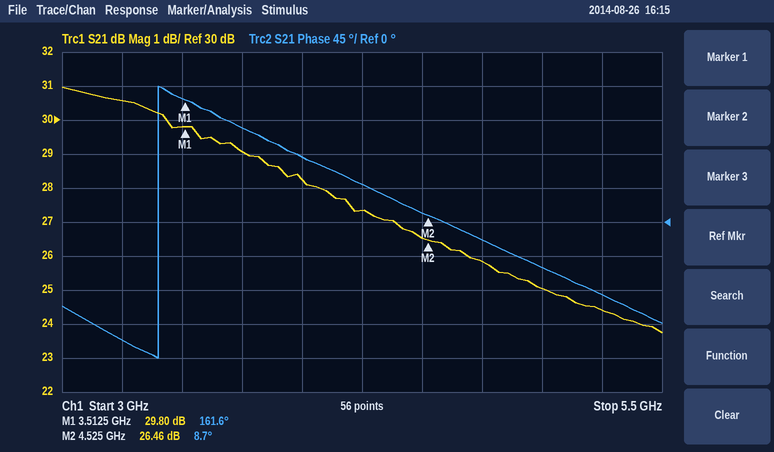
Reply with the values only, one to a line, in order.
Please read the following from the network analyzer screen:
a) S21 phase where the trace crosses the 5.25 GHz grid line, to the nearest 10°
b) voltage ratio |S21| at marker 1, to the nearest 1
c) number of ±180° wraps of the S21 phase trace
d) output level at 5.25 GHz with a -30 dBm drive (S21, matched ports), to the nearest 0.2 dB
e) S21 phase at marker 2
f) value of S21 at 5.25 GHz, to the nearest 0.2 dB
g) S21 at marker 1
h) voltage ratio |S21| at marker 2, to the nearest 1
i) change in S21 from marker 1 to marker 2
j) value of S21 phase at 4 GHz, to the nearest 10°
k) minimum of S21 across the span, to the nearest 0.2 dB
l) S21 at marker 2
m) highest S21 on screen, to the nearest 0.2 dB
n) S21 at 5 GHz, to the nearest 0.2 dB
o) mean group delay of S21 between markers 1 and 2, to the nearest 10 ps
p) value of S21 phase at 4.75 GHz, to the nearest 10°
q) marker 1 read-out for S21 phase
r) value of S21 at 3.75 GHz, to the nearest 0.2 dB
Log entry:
-100°
31
1
-5.6 dBm
8.7°
24.4 dB
29.80 dB
21
-3.34 dB
90°
23.8 dB
26.46 dB
31.0 dB
25.0 dB
420 ps
-20°
161.6°
29.0 dB
